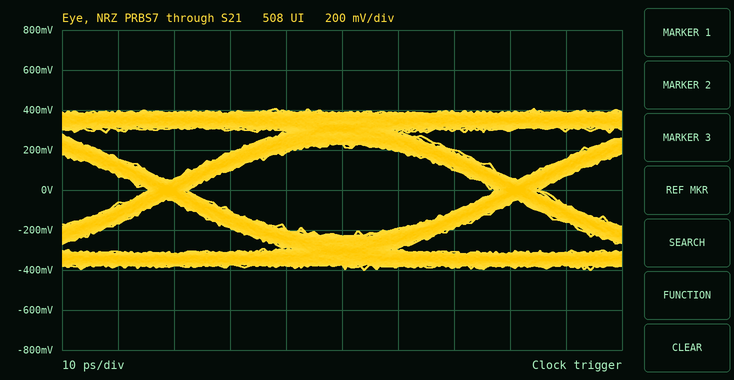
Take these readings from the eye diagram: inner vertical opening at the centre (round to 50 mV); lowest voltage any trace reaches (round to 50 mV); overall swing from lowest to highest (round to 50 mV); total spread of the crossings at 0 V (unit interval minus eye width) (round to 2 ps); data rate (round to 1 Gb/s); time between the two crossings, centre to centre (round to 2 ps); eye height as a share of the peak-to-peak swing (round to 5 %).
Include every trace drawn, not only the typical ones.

450 mV
-400 mV
800 mV
8 ps
16 Gb/s
62 ps
55 %
